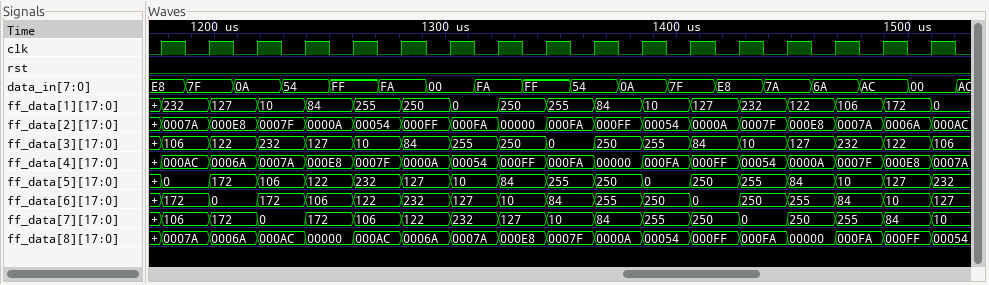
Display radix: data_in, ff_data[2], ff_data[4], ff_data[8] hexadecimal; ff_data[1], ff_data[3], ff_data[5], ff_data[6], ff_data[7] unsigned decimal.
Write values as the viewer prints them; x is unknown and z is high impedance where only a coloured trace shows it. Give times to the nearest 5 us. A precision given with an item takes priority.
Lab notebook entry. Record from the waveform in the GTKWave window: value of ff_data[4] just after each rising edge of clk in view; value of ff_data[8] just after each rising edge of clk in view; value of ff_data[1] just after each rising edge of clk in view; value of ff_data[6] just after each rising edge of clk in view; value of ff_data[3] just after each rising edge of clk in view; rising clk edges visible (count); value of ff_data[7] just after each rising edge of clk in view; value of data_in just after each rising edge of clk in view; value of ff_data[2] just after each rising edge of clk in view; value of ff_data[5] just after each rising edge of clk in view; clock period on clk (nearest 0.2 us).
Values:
000AC, 0006A, 0007A, 000E8, 0007F, 0000A, 00054, 000FF, 000FA, 00000, 000FA, 000FF, 00054, 0000A, 0007F, 000E8, 0007A
0007A, 0006A, 000AC, 00000, 000AC, 0006A, 0007A, 000E8, 0007F, 0000A, 00054, 000FF, 000FA, 00000, 000FA, 000FF, 00054
232, 127, 10, 84, 255, 250, 0, 250, 255, 84, 10, 127, 232, 122, 106, 172, 0
172, 0, 172, 106, 122, 232, 127, 10, 84, 255, 250, 0, 250, 255, 84, 10, 127
106, 122, 232, 127, 10, 84, 255, 250, 0, 250, 255, 84, 10, 127, 232, 122, 106
17
106, 172, 0, 172, 106, 122, 232, 127, 10, 84, 255, 250, 0, 250, 255, 84, 10
E8, 7F, 0A, 54, FF, FA, 00, FA, FF, 54, 0A, 7F, E8, 7A, 6A, AC, 00
0007A, 000E8, 0007F, 0000A, 00054, 000FF, 000FA, 00000, 000FA, 000FF, 00054, 0000A, 0007F, 000E8, 0007A, 0006A, 000AC
0, 172, 106, 122, 232, 127, 10, 84, 255, 250, 0, 250, 255, 84, 10, 127, 232
20.8 us
